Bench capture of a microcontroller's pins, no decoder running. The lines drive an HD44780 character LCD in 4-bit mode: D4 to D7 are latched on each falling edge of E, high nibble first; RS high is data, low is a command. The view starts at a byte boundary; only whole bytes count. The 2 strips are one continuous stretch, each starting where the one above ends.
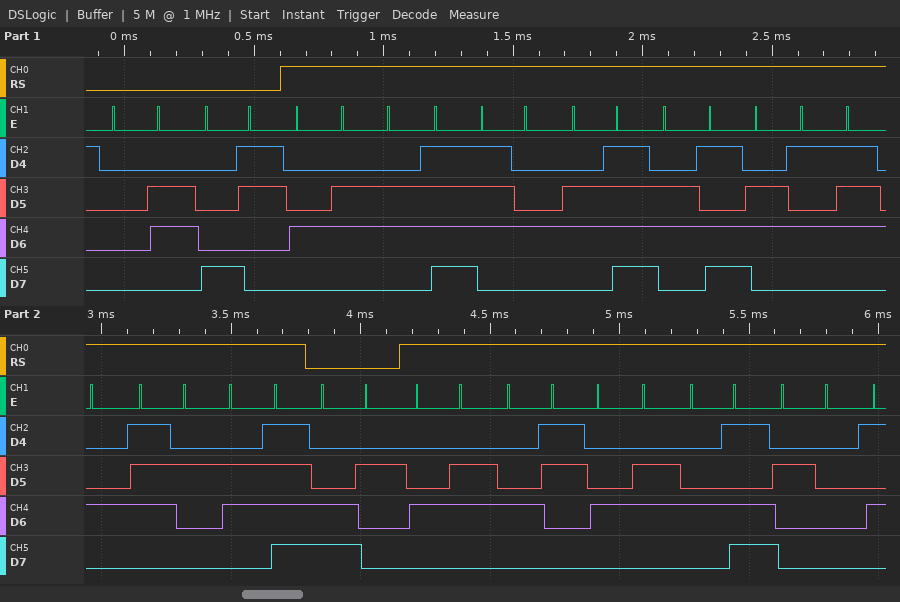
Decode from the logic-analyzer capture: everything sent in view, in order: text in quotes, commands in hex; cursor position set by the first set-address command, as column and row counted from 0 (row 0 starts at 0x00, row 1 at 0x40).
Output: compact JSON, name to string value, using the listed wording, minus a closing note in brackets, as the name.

{"everything sent in view, in order: text in quotes, commands in hex": "0x06 0x83 \"Fotometro\" 0xC2 \"FCFM \"", "cursor position set by the first set-address command, as column and row counted from 0": "column 3, row 0"}
